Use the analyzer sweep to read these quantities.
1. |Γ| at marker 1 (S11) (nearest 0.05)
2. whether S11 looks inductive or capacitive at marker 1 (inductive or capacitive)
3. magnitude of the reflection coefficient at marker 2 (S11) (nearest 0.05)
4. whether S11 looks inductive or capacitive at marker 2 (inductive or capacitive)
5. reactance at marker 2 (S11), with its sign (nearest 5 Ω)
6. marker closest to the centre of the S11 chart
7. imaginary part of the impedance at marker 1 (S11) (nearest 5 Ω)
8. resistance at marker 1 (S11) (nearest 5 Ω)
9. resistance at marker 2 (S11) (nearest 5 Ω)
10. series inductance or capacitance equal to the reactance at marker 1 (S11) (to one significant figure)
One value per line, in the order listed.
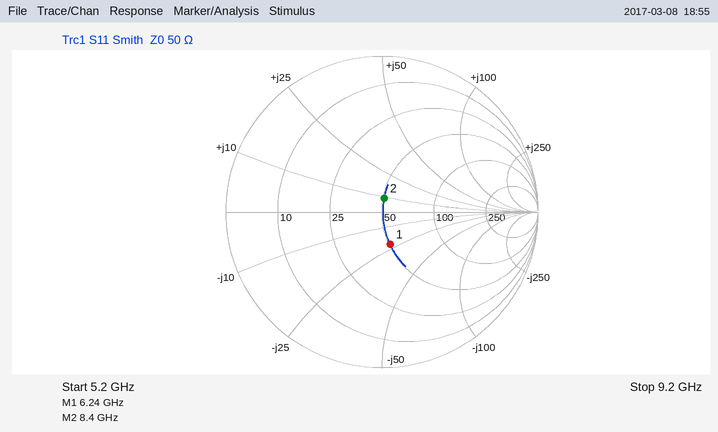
0.20
capacitive
0.10
inductive
+10 Ω
marker 2
-20 Ω
50 Ω
50 Ω
1 pF
